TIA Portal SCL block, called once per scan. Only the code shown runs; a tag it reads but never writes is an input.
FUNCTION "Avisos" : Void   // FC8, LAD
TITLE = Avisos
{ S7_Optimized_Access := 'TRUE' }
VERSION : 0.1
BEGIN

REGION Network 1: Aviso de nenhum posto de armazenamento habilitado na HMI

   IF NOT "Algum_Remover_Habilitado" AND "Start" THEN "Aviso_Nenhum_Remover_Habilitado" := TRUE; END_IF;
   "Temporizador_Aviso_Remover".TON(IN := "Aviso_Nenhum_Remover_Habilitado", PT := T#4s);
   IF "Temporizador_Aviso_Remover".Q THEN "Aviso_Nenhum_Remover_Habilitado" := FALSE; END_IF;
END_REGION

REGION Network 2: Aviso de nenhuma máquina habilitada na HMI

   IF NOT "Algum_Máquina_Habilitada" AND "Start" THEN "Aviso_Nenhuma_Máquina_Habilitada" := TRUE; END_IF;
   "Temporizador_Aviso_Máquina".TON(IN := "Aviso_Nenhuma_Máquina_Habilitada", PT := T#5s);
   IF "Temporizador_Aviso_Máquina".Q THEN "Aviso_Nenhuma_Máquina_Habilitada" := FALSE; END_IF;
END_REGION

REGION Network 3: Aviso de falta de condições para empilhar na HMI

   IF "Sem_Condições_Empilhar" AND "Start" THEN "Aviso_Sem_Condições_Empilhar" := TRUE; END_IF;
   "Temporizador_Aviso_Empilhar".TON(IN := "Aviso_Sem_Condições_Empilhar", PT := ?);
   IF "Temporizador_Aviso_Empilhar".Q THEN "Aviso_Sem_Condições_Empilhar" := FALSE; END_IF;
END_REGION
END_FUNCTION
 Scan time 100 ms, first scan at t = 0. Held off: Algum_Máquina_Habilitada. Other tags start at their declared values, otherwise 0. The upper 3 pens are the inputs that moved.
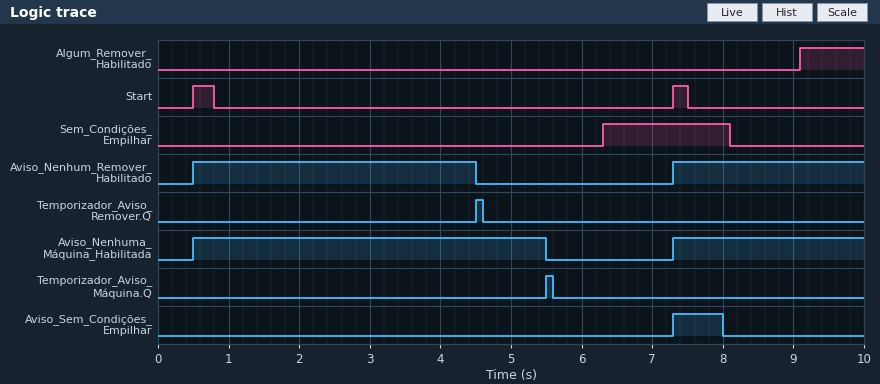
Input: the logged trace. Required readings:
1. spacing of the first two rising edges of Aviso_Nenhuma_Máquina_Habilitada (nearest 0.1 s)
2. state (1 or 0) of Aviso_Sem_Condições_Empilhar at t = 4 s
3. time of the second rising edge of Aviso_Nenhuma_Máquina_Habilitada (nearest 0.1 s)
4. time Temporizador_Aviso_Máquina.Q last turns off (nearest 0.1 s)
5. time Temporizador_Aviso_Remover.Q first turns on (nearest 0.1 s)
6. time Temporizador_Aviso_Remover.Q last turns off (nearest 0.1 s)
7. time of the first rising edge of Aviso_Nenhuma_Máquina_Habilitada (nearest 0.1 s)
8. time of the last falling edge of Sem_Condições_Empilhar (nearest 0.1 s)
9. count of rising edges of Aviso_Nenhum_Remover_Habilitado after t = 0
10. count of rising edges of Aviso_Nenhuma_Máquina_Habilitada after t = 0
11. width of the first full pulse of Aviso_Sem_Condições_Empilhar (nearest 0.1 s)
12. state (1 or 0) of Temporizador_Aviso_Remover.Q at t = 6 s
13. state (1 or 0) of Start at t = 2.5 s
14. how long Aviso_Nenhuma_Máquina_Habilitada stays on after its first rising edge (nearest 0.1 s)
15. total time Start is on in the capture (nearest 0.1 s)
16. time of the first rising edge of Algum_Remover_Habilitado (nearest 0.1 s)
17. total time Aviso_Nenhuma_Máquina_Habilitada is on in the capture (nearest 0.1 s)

6.8 s
0
7.3 s
5.6 s
4.5 s
4.6 s
0.5 s
8.1 s
2
2
0.7 s
0
0
5.0 s
0.5 s
9.1 s
7.7 s
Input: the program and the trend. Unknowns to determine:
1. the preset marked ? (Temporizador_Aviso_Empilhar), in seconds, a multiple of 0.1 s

0.7 s
